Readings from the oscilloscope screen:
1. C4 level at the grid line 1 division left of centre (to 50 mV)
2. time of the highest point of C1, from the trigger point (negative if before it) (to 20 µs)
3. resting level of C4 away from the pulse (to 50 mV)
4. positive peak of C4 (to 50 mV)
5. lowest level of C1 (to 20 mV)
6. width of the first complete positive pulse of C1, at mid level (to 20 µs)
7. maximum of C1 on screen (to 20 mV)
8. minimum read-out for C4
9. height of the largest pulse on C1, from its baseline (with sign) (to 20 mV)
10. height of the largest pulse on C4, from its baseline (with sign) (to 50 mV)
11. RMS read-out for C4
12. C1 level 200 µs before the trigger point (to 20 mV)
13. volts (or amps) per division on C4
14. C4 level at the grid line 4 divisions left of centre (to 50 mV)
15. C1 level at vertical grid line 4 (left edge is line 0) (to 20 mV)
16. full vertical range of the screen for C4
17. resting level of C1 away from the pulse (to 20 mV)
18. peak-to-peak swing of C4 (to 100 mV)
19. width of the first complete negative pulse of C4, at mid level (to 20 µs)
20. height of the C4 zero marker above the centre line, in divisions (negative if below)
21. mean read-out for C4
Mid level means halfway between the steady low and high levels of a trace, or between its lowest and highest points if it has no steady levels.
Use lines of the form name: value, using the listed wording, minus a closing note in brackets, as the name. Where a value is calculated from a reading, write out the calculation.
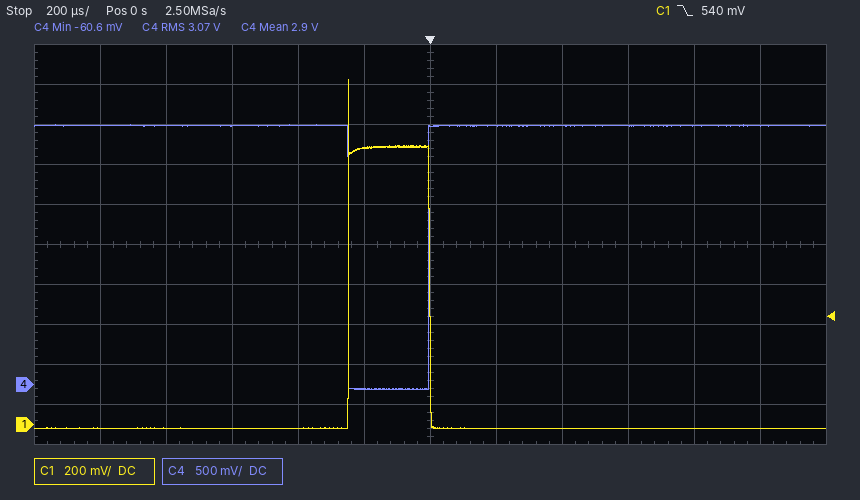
C4 level at the grid line 1 division left of centre: -50 mV
time of the highest point of C1, from the trigger point (negative if before it): -240 µs
resting level of C4 away from the pulse: 3.25 V
positive peak of C4: 3.25 V
lowest level of C1: -20 mV
width of the first complete positive pulse of C1, at mid level: 240 µs
maximum of C1 on screen: 1.72 V
minimum read-out for C4: -60.6 mV
height of the largest pulse on C1, from its baseline (with sign): 1.72 V − (-20 mV) = +1.74 V
height of the largest pulse on C4, from its baseline (with sign): -3.30 V
RMS read-out for C4: 3.07 V
C1 level 200 µs before the trigger point: 1.38 V
volts (or amps) per division on C4: 500 mV
C4 level at the grid line 4 divisions left of centre: 3.25 V
C1 level at vertical grid line 4 (left edge is line 0): -20 mV
full vertical range of the screen for C4: 5 V
resting level of C1 away from the pulse: -20 mV
peak-to-peak swing of C4: 3.30 V
width of the first complete negative pulse of C4, at mid level: 240 µs
height of the C4 zero marker above the centre line, in divisions: -3.5 div
mean read-out for C4: 2.9 V
